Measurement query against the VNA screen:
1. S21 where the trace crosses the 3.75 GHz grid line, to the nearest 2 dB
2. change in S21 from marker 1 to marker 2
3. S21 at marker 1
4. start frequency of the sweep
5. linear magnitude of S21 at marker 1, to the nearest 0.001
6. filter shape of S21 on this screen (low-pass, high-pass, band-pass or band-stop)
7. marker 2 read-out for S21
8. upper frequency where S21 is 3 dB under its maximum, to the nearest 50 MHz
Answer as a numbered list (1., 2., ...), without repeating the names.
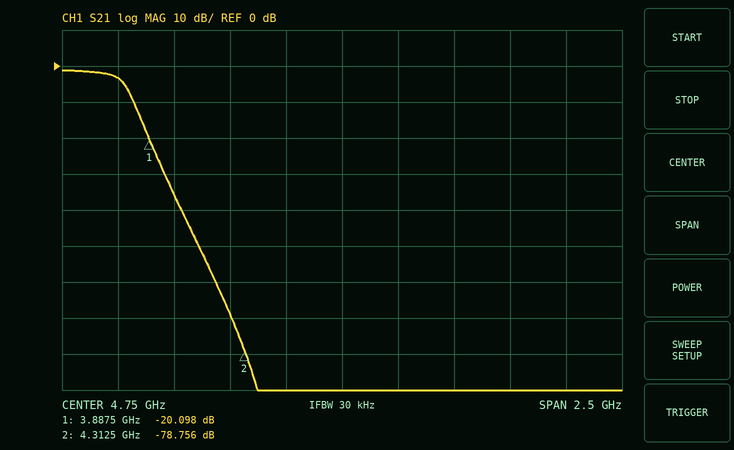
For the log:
1. -4 dB
2. -58.658 dB
3. -20.098 dB
4. 3.5 GHz
5. 0.099
6. low-pass
7. -78.756 dB
8. 3.75 GHz
